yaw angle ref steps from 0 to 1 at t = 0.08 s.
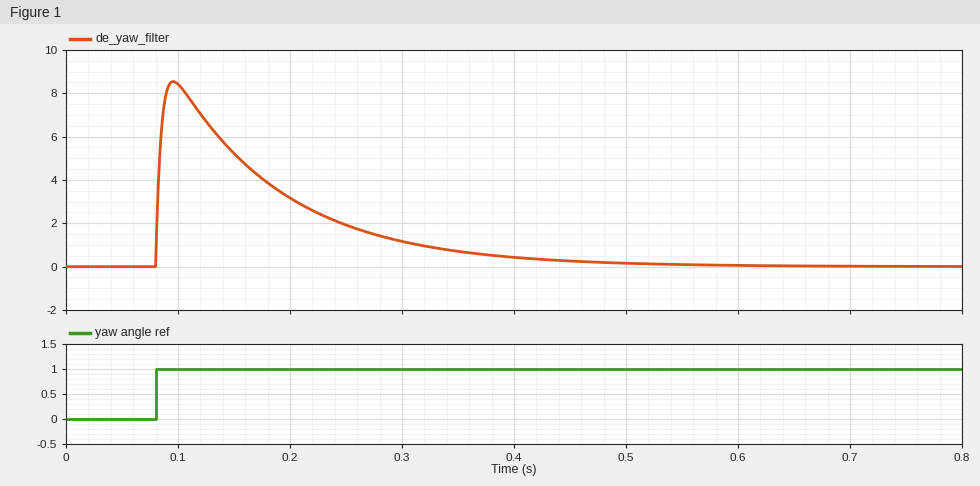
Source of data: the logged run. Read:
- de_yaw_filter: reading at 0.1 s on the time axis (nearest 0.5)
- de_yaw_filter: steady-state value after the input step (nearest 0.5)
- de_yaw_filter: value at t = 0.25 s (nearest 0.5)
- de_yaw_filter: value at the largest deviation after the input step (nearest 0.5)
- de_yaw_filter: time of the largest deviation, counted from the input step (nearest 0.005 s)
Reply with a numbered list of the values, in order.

1. 8.5
2. 0.0
3. 2.0
4. 8.5
5. 0.015 s
